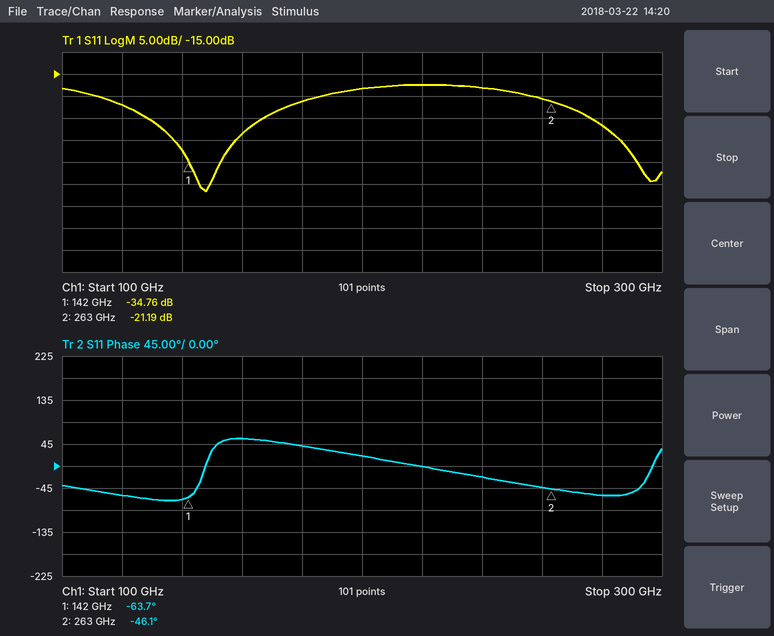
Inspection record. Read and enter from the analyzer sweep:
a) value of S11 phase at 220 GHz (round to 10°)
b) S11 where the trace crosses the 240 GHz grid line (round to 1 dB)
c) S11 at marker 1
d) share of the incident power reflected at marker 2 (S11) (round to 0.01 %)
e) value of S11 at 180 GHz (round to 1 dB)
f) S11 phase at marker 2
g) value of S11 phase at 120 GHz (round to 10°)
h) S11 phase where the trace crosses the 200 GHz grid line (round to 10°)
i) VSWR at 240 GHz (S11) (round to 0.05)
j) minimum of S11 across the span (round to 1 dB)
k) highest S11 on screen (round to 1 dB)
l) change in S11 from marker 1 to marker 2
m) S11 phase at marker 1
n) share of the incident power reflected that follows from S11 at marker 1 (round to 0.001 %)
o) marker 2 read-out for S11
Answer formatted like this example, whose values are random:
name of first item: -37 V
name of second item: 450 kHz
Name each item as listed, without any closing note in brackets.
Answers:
value of S11 phase at 220 GHz: 0°
S11 where the trace crosses the 240 GHz grid line: -18 dB
S11 at marker 1: -34.76 dB
share of the incident power reflected at marker 2 (S11): 0.76 %
value of S11 at 180 GHz: -21 dB
S11 phase at marker 2: -46.1°
value of S11 phase at 120 GHz: -60°
S11 phase where the trace crosses the 200 GHz grid line: 20°
VSWR at 240 GHz (S11): 1.30
minimum of S11 across the span: -42 dB
highest S11 on screen: -17 dB
change in S11 from marker 1 to marker 2: 13.57 dB
S11 phase at marker 1: -63.7°
share of the incident power reflected that follows from S11 at marker 1: 0.033 %
marker 2 read-out for S11: -21.19 dB
